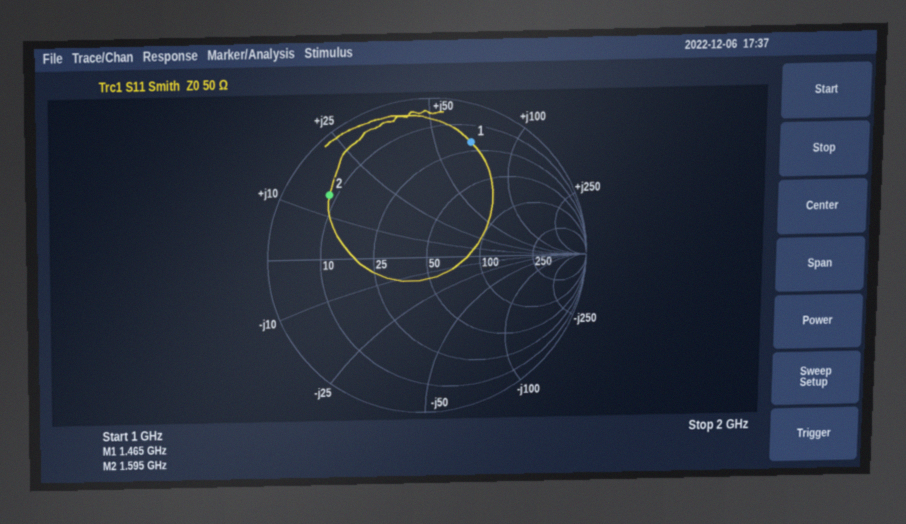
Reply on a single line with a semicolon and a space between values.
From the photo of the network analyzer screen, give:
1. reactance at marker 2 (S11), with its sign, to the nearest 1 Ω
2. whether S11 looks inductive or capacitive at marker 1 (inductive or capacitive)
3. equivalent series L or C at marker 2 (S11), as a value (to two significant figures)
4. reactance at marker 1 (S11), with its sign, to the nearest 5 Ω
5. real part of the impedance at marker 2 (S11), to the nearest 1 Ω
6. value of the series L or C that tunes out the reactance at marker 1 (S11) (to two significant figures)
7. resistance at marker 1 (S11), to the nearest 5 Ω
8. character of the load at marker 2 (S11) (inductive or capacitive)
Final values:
+15 Ω; inductive; 1.5 nH; +70 Ω; 8 Ω; 1.6 pF; 20 Ω; inductive
